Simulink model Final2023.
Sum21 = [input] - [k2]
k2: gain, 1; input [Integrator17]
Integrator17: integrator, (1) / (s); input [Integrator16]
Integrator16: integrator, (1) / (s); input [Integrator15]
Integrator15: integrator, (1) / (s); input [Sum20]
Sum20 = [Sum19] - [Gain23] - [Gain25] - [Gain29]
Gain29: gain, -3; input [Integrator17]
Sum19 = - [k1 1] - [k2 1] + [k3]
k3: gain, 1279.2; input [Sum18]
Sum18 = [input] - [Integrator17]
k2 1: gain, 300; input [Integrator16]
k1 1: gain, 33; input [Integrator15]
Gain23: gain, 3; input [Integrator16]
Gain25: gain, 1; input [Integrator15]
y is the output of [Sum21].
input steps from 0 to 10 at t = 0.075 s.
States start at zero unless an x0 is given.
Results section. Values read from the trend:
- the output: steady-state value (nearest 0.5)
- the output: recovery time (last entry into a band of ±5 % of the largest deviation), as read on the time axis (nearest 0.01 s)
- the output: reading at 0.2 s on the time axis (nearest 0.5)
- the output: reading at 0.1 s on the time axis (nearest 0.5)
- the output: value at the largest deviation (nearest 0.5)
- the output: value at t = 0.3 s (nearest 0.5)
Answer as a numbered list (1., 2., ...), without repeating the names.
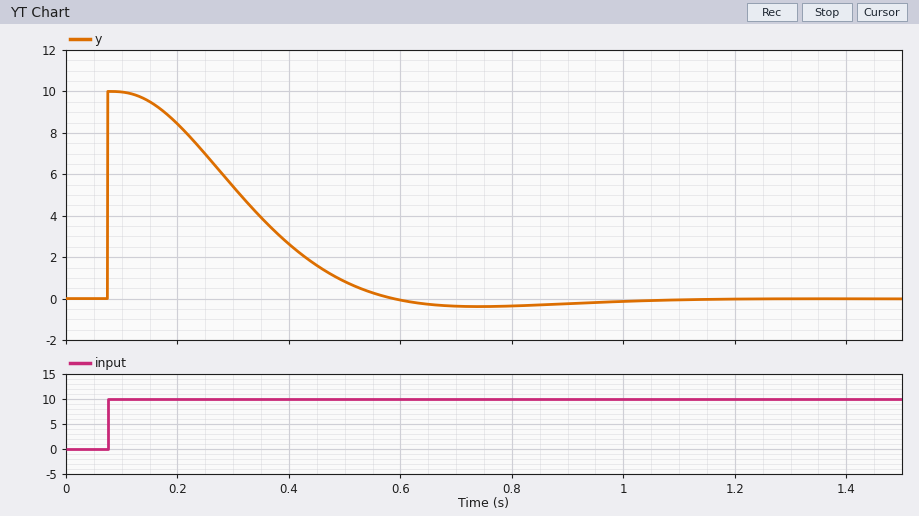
1. 0.0
2. 0.53 s
3. 8.5
4. 10.0
5. 10.0
6. 5.5
